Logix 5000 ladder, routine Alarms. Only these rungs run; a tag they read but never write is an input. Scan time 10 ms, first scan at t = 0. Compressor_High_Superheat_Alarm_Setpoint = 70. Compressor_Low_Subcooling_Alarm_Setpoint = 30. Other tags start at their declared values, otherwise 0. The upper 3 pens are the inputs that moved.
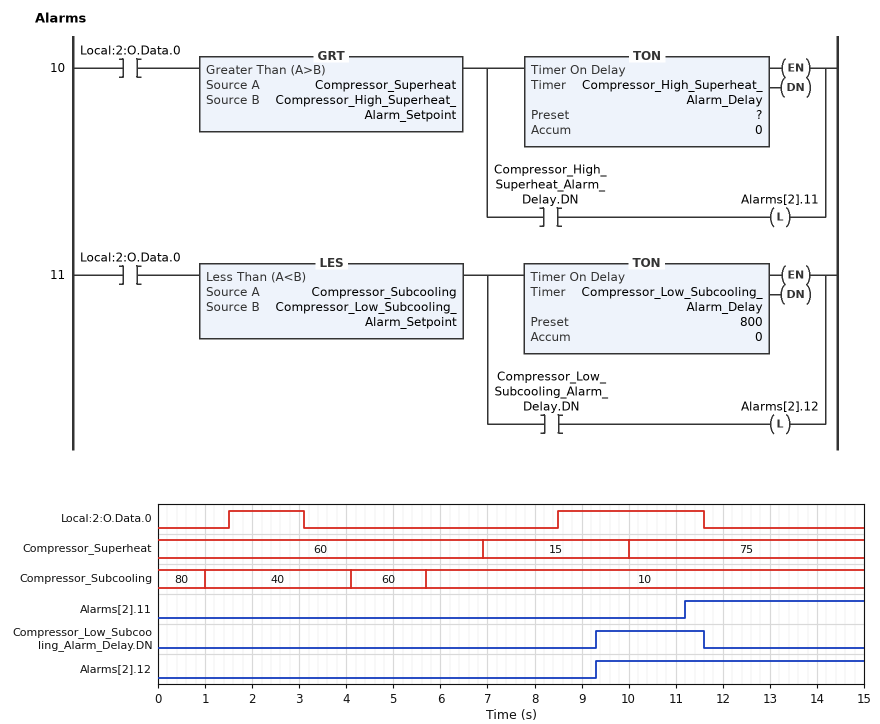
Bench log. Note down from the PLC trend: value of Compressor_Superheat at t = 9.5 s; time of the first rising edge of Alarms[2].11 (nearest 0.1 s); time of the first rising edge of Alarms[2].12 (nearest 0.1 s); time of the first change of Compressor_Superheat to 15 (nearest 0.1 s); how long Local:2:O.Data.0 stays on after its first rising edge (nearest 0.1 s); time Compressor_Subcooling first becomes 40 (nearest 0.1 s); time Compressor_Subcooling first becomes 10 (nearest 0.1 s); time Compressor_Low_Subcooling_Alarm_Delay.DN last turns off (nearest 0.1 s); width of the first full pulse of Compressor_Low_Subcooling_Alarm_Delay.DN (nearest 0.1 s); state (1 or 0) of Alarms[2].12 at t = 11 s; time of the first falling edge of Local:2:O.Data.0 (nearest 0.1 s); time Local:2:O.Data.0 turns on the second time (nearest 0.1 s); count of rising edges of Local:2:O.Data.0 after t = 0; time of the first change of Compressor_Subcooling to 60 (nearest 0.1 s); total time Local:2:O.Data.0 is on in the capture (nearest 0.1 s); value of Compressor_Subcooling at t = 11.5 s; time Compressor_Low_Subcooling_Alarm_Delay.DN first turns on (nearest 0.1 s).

15
11.2 s
9.3 s
6.9 s
1.6 s
1.0 s
5.7 s
11.6 s
2.3 s
1
3.1 s
8.5 s
2
4.1 s
4.7 s
10
9.3 s
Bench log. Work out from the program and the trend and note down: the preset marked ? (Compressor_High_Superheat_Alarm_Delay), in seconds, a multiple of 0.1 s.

1.2 s
